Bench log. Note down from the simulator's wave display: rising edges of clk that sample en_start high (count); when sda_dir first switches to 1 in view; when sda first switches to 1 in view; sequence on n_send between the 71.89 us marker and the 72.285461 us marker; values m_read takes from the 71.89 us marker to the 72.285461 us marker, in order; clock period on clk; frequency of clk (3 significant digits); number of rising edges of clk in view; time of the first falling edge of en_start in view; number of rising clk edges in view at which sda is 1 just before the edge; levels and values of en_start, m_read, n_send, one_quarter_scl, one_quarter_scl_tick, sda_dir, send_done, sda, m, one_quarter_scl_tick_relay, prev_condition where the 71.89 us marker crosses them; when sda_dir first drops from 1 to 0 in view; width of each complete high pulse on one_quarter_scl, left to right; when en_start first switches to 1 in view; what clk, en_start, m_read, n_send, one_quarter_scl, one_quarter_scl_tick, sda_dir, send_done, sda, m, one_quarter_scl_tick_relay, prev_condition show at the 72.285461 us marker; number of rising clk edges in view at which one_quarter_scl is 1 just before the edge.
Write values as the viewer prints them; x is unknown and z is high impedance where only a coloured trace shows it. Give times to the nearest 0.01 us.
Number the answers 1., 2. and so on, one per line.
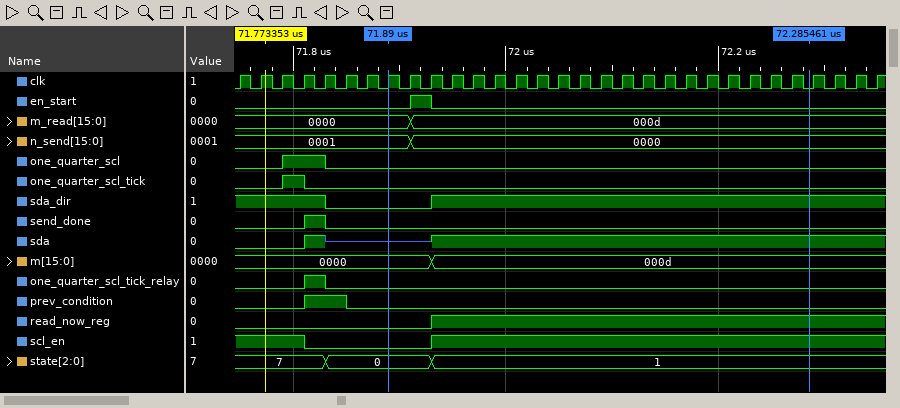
1. 1
2. 71.93 us
3. 71.81 us
4. 0001, 0000
5. 0000, 000d
6. 0.02 us
7. 50.0 MHz
8. 31
9. 71.93 us
10. 22
11. en_start=0, m_read=0000, n_send=0001, one_quarter_scl=0, one_quarter_scl_tick=0, sda_dir=0, send_done=0, sda=z, m=0000, one_quarter_scl_tick_relay=0, prev_condition=0
12. 71.83 us
13. 0.04 us
14. 71.91 us
15. clk=0, en_start=0, m_read=000d, n_send=0000, one_quarter_scl=0, one_quarter_scl_tick=0, sda_dir=1, send_done=0, sda=1, m=000d, one_quarter_scl_tick_relay=0, prev_condition=0
16. 2
